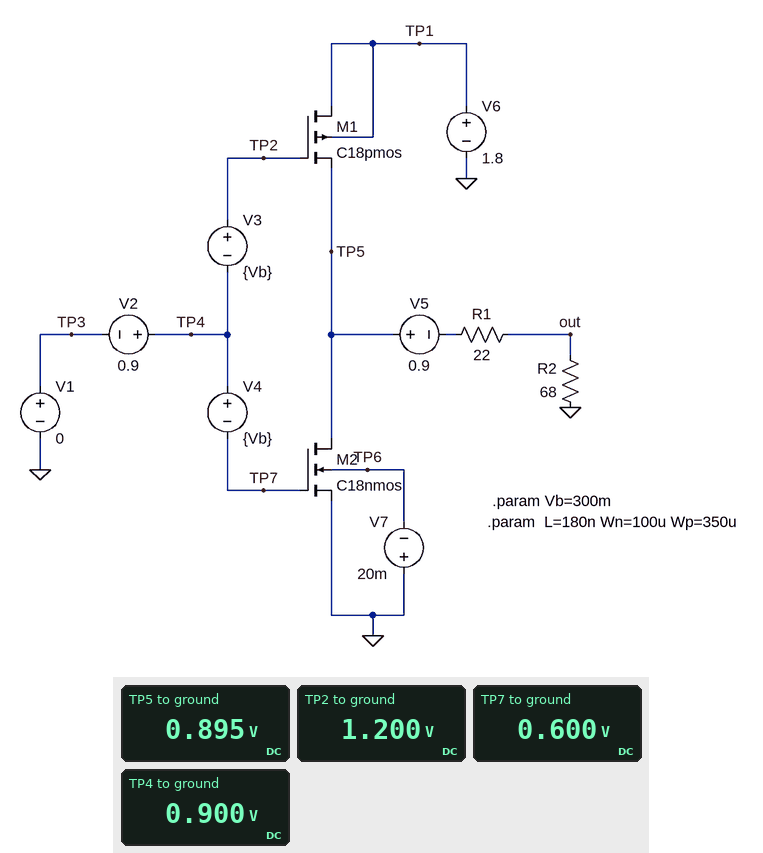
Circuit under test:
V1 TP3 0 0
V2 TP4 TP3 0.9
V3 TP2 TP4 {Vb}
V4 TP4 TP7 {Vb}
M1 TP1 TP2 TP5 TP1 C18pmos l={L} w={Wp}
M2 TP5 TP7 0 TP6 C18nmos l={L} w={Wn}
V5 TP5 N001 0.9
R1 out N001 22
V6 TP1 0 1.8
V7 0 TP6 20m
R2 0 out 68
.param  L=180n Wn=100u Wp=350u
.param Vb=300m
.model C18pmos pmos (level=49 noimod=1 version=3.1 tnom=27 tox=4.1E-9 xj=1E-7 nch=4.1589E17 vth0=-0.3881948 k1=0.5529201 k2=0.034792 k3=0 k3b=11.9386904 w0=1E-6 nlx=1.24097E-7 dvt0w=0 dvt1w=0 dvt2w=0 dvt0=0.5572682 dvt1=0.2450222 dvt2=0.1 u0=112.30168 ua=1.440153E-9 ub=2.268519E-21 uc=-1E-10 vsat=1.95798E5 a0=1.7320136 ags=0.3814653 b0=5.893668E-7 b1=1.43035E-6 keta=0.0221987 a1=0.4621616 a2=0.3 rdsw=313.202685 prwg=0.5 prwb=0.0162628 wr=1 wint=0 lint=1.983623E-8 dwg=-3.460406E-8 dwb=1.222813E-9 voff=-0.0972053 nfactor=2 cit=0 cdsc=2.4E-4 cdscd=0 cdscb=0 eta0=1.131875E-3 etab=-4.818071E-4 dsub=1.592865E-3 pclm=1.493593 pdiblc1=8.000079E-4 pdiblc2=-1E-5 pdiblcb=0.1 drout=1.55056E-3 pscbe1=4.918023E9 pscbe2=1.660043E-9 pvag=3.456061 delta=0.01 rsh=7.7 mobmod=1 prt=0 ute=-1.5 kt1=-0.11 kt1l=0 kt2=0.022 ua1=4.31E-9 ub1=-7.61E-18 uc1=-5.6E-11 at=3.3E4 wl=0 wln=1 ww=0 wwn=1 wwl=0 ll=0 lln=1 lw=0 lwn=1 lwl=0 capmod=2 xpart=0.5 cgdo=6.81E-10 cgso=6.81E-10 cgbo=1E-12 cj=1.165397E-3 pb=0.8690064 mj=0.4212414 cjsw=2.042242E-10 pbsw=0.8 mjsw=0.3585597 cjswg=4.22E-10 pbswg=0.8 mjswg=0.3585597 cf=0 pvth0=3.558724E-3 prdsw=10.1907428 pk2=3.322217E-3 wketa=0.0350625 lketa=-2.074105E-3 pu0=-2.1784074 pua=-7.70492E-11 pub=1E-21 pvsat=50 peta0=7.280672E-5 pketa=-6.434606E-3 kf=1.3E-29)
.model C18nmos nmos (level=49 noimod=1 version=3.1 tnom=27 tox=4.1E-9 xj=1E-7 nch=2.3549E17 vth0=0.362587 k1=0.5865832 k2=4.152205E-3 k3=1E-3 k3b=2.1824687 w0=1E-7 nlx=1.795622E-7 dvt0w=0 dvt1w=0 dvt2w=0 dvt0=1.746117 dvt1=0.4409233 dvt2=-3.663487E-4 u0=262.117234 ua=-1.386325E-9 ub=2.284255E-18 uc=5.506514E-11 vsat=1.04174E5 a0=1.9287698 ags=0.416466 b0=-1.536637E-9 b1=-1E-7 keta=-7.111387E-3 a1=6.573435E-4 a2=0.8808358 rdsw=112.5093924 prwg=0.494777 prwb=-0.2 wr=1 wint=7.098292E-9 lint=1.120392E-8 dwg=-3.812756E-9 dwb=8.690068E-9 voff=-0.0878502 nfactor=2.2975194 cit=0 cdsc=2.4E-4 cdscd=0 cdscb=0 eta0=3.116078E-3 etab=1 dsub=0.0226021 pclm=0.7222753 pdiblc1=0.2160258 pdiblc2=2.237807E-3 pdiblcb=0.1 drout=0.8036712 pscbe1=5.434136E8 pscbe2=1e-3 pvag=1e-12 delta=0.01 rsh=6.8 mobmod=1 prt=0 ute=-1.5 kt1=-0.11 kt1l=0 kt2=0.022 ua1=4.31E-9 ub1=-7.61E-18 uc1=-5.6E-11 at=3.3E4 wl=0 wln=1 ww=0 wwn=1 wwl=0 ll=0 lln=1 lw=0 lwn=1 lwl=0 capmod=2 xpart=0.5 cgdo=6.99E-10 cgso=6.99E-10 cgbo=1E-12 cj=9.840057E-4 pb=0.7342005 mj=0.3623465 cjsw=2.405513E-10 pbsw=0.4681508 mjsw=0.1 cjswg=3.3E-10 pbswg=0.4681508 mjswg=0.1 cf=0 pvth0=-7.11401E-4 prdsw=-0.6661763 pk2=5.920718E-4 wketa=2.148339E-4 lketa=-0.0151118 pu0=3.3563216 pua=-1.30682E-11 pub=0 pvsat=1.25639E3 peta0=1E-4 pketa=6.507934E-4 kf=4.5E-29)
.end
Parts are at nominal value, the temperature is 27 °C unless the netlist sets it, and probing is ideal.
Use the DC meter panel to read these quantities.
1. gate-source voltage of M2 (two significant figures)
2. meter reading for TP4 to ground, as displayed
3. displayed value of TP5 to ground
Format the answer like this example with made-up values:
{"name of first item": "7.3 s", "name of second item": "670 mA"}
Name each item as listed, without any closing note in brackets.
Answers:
{"gate-source voltage of M2": "600 mV", "meter reading for TP4 to ground, as displayed": "0.900 V", "displayed value of TP5 to ground": "0.895 V"}
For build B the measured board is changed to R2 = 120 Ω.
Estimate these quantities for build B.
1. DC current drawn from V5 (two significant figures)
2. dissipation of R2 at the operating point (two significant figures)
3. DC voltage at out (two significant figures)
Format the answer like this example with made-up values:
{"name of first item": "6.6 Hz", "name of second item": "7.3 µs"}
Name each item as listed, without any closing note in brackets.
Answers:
{"DC current drawn from V5": "58 µA", "dissipation of R2 at the operating point": "400 nW", "DC voltage at out": "-6.9 mV"}
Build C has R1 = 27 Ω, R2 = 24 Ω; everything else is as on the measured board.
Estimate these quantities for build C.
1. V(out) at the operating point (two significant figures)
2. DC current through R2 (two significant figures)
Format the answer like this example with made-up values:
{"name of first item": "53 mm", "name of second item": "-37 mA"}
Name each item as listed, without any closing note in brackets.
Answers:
{"V(out) at the operating point": "-1.4 mV", "DC current through R2": "60 µA"}
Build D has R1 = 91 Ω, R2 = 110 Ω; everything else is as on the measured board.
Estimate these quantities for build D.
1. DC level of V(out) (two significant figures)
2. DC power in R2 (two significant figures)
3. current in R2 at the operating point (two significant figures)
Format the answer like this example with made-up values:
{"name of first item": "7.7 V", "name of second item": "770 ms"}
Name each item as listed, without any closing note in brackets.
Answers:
{"DC level of V(out)": "-6.2 mV", "DC power in R2": "350 nW", "current in R2 at the operating point": "57 µA"}
